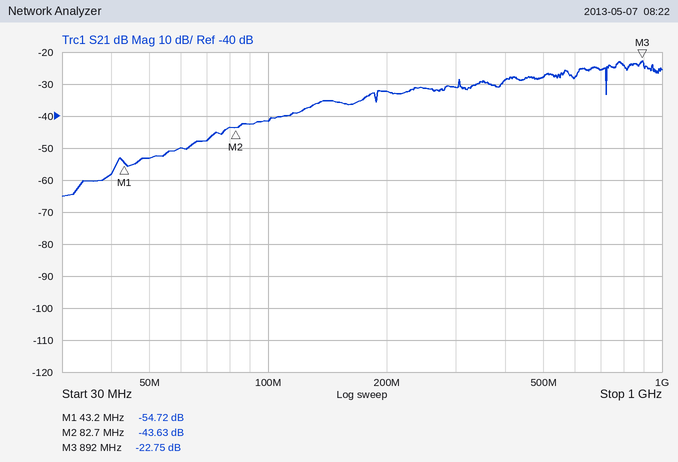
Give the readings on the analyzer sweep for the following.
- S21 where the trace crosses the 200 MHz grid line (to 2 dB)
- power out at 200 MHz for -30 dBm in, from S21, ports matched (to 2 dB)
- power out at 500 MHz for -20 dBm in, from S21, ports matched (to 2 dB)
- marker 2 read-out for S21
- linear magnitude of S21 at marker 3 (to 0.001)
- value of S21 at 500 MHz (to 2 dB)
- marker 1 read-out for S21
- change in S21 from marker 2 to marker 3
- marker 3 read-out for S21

-32 dB
-62 dBm
-48 dBm
-43.63 dB
0.073
-28 dB
-54.72 dB
20.88 dB
-22.75 dB
